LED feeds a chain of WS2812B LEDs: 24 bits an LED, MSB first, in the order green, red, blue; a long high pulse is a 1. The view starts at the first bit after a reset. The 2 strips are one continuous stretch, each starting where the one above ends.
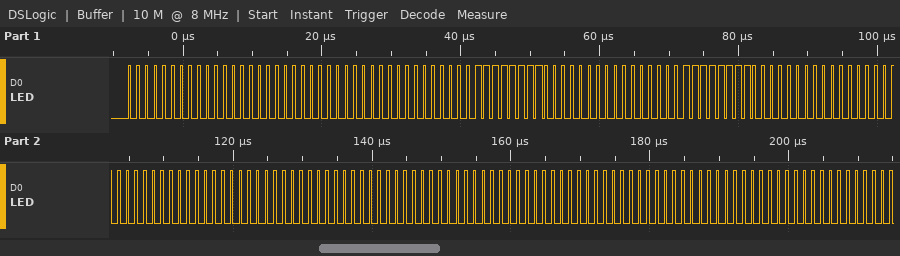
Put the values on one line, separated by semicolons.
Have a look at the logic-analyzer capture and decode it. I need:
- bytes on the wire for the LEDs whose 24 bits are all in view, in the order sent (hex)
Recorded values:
00 00 00 00 00 FF 00 00 FF 00 00 00 00 00 00 00 00 00 00 00 00
